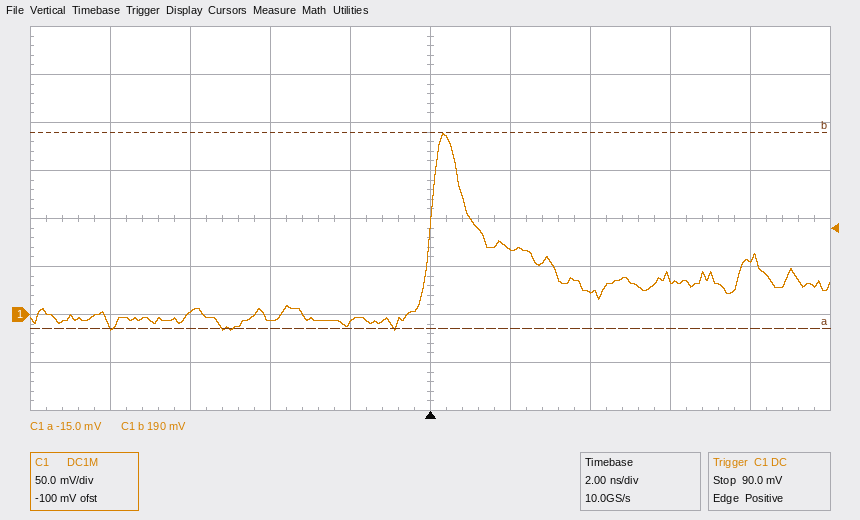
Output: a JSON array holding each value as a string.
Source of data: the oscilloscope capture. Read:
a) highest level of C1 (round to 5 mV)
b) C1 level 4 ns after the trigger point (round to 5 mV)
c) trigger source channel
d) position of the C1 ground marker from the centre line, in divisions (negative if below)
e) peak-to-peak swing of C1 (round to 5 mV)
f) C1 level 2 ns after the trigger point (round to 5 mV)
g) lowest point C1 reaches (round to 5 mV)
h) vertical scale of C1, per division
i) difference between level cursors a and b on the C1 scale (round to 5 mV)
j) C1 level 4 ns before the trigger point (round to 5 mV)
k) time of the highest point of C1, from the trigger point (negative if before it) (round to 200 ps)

["190 mV", "25 mV", "C1", "-2.0 div", "205 mV", "70 mV", "-15 mV", "50 mV", "205 mV", "-5 mV", "+400 ps"]
